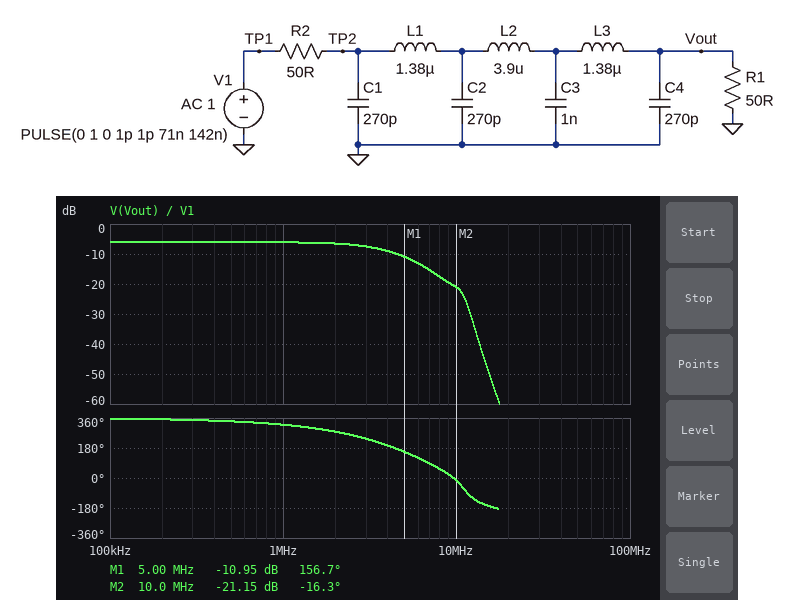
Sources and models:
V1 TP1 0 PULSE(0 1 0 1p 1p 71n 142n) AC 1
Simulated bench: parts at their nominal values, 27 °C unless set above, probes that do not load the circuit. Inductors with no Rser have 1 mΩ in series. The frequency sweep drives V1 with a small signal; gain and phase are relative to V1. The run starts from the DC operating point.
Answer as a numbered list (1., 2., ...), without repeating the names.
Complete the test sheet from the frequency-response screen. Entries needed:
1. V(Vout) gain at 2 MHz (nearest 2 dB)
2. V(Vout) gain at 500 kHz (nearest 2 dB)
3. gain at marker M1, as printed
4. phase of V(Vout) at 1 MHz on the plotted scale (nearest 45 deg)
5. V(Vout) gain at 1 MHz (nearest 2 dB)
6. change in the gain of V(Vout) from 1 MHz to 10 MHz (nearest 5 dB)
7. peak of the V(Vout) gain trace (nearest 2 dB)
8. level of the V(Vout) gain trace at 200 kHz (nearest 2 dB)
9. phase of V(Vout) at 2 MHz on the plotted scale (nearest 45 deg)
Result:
1. -6 dB
2. -6 dB
3. -10.95 dB
4. 315 deg
5. -6 dB
6. -15 dB
7. -6 dB
8. -6 dB
9. 270 deg
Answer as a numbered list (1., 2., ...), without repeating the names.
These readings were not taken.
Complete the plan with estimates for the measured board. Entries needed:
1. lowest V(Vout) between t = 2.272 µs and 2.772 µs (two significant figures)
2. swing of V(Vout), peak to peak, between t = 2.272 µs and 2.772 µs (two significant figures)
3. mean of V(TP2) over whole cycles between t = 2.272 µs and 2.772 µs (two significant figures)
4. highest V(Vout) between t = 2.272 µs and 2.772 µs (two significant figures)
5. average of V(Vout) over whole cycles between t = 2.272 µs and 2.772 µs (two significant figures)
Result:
1. 140 mV
2. 210 mV
3. 250 mV
4. 360 mV
5. 250 mV
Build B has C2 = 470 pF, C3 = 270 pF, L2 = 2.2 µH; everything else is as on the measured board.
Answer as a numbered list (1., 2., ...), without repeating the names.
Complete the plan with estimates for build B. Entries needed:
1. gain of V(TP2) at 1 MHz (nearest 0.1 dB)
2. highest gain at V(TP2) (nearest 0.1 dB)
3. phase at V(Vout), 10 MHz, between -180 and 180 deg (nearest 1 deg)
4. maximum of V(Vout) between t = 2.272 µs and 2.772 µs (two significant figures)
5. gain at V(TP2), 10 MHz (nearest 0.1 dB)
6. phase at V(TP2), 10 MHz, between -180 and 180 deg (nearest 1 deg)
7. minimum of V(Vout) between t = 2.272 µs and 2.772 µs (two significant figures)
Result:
1. -5.5 dB
2. -0.9 dB
3. 44 deg
4. 530 mV
5. -1.4 dB
6. 6 deg
7. -28 mV
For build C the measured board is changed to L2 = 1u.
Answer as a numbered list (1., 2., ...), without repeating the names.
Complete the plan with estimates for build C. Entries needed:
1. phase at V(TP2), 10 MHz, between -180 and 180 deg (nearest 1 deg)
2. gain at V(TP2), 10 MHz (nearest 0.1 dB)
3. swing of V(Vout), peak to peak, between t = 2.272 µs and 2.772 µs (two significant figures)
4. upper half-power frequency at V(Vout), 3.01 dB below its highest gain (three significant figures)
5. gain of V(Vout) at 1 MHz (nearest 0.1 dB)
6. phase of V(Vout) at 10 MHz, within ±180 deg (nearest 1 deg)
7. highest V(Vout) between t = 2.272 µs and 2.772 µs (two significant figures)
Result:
1. -32 deg
2. -1.7 dB
3. 410 mV
4. 6.66 MHz
5. -6.0 dB
6. 49 deg
7. 460 mV
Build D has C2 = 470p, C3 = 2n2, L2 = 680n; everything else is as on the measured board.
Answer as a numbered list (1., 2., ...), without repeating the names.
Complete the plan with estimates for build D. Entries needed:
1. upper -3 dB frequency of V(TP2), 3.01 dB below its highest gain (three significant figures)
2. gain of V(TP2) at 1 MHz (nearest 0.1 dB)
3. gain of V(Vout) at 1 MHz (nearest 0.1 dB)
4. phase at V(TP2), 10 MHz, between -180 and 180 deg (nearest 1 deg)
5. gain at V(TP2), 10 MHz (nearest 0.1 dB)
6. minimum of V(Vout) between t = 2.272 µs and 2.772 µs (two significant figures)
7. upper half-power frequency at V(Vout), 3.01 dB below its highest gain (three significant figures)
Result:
1. 16.9 MHz
2. -7.7 dB
3. -6.4 dB
4. -41 deg
5. -2.6 dB
6. 150 mV
7. 3.48 MHz
